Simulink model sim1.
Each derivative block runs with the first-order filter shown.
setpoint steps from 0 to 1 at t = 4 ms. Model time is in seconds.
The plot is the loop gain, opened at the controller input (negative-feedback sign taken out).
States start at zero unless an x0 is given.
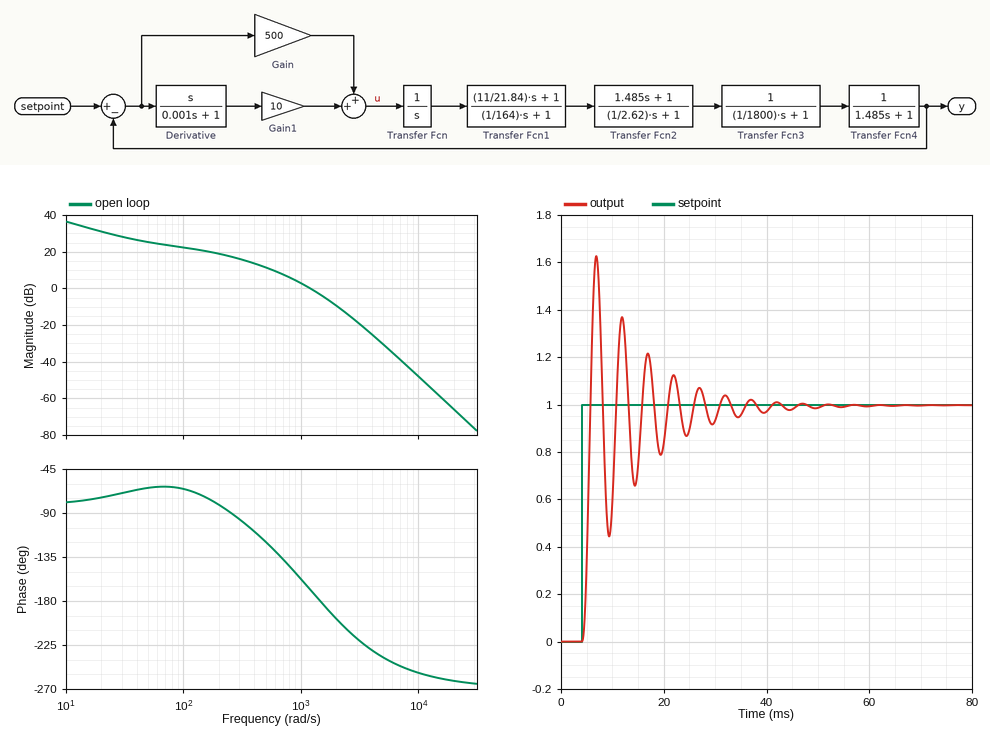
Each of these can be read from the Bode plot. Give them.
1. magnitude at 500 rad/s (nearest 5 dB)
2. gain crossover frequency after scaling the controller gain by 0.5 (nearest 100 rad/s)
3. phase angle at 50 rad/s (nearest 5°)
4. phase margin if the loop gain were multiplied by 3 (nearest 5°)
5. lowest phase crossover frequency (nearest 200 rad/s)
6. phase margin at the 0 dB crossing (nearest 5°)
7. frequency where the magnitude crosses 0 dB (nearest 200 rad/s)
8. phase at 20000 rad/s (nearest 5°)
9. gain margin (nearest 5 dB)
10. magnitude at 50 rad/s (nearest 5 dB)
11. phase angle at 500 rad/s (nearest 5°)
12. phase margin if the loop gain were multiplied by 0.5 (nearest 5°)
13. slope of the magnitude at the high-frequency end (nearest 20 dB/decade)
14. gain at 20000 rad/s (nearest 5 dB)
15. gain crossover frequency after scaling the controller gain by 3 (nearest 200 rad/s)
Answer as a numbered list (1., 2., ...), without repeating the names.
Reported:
1. 10 dB
2. 800 rad/s
3. -65°
4. -20°
5. 1400 rad/s
6. 10°
7. 1200 rad/s
8. -260°
9. 5 dB
10. 25 dB
11. -120°
12. 35°
13. -60 dB/decade
14. -65 dB
15. 2000 rad/s
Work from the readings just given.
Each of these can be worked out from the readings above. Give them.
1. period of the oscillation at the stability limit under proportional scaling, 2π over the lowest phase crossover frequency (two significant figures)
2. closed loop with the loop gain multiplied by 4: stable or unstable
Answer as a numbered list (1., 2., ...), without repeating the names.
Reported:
1. 0.0045 s
2. unstable
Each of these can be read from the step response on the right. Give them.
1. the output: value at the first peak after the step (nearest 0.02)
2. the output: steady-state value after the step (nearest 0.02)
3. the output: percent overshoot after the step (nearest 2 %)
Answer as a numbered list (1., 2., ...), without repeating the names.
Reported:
1. 1.62
2. 1.00
3. 62 %
